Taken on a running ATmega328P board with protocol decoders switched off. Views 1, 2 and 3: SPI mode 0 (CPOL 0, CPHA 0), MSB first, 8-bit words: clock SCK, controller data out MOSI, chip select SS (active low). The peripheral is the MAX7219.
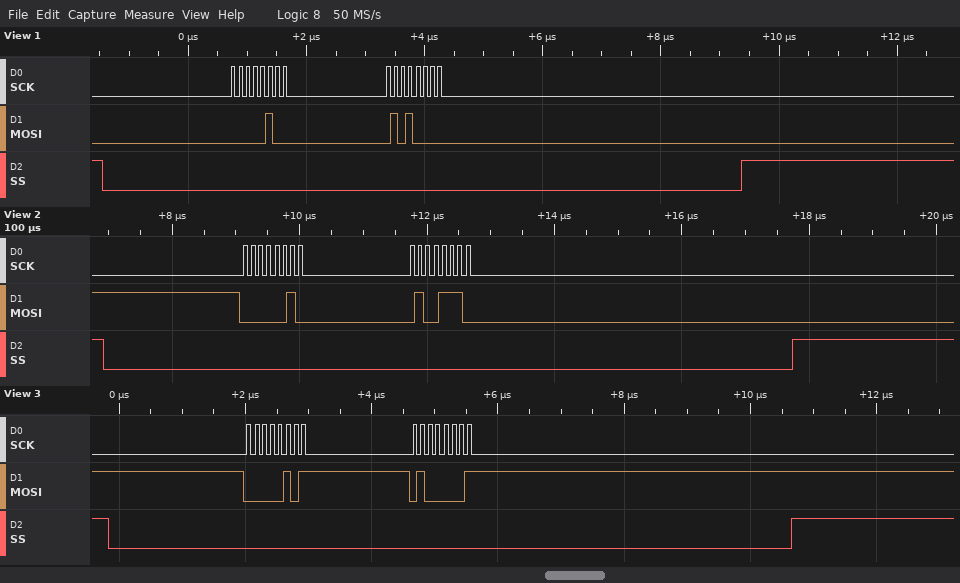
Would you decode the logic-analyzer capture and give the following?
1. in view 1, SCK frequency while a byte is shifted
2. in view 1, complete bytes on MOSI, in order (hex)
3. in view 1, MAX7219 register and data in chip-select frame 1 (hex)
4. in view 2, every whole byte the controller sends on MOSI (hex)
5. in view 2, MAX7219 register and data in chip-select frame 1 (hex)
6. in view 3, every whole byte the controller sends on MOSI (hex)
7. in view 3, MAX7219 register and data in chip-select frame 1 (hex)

8 MHz
0x04 0x50
register 0x4, data 0x50
02 4E
register 0x2, data 0x4E
05 41
register 0x5, data 0x41
